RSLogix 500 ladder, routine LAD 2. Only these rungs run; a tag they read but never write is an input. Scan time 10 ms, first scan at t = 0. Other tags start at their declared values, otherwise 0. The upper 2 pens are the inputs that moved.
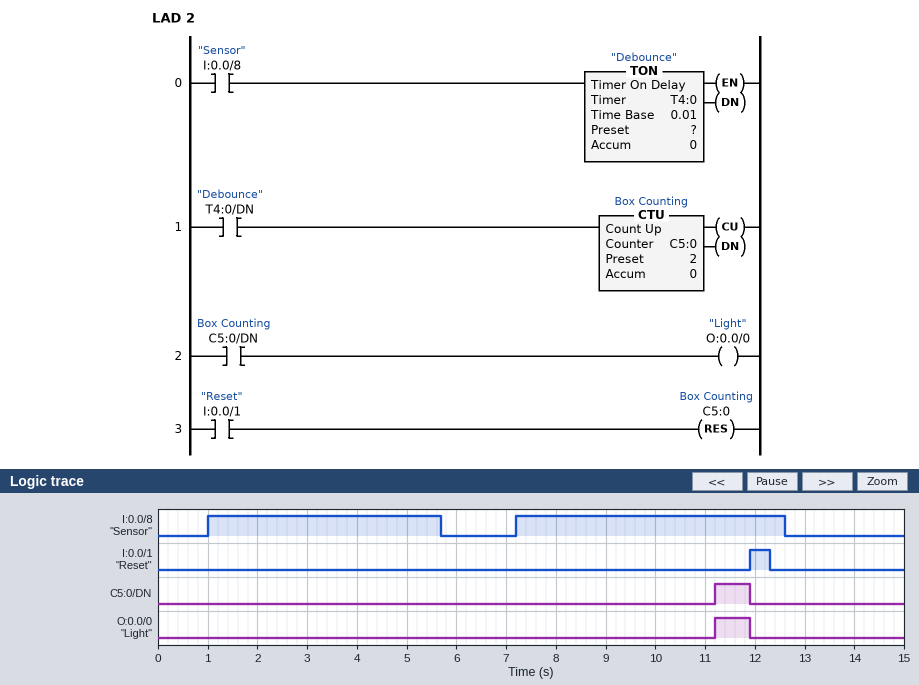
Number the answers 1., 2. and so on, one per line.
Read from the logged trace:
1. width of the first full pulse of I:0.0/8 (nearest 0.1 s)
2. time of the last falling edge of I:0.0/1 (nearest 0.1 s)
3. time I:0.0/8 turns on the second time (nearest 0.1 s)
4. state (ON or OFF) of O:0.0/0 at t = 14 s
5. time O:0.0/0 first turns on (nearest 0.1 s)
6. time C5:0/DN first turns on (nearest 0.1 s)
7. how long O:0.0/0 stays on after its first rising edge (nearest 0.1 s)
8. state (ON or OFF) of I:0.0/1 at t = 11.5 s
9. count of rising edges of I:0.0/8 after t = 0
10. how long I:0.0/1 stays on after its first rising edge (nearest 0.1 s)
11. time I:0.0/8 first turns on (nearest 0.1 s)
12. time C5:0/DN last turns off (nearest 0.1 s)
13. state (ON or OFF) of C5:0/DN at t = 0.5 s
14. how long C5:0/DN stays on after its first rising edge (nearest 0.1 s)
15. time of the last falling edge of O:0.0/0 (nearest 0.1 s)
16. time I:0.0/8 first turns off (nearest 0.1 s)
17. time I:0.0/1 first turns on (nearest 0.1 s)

1. 4.7 s
2. 12.3 s
3. 7.2 s
4. OFF
5. 11.2 s
6. 11.2 s
7. 0.7 s
8. OFF
9. 2
10. 0.4 s
11. 1.0 s
12. 11.9 s
13. OFF
14. 0.7 s
15. 11.9 s
16. 5.7 s
17. 11.9 s
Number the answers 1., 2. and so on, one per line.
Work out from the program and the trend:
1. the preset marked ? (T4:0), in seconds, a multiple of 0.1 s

1. 4.0 s
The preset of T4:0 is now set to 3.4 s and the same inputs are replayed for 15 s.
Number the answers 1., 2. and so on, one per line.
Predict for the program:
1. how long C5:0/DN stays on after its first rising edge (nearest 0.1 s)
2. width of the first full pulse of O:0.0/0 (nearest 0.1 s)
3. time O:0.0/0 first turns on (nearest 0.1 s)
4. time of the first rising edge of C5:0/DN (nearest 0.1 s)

1. 1.3 s
2. 1.3 s
3. 10.6 s
4. 10.6 s
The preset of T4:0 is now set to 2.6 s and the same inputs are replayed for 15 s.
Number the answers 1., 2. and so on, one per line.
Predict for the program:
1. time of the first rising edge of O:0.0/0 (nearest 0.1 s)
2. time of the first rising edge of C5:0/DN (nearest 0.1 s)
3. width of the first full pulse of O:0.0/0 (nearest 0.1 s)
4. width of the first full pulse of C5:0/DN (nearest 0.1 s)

1. 9.8 s
2. 9.8 s
3. 2.1 s
4. 2.1 s
